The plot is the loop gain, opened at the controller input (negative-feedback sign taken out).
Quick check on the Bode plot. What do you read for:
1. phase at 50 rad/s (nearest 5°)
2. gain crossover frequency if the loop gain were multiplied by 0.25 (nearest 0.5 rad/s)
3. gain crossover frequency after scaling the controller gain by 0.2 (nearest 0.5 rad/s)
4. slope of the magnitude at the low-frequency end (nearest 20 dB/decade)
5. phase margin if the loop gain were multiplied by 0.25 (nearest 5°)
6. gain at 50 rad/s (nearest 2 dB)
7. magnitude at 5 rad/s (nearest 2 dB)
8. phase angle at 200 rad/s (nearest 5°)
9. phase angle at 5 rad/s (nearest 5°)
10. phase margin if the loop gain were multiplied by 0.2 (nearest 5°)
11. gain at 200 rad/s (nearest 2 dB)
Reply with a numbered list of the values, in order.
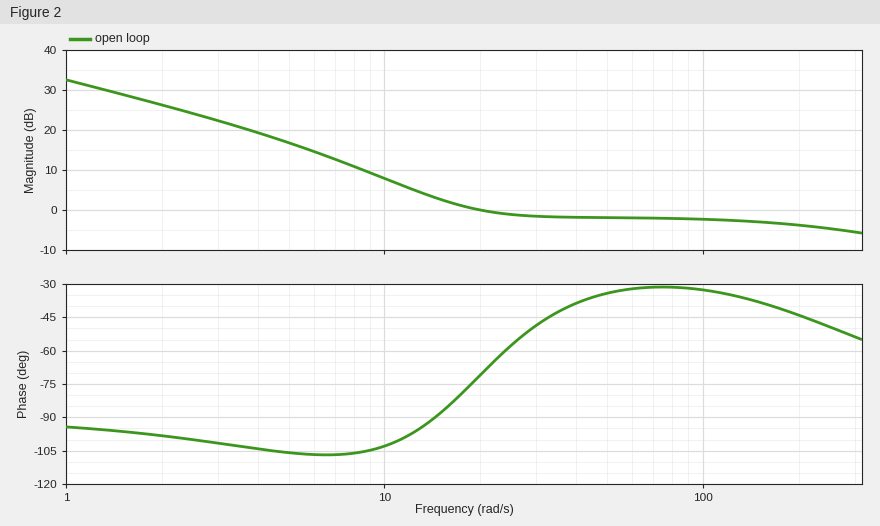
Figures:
1. -35°
2. 7.5 rad/s
3. 6.5 rad/s
4. -20 dB/decade
5. 75°
6. -2 dB
7. 16 dB
8. -45°
9. -105°
10. 75°
11. -4 dB
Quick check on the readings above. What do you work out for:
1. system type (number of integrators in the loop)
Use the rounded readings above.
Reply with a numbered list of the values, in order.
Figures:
1. 1
